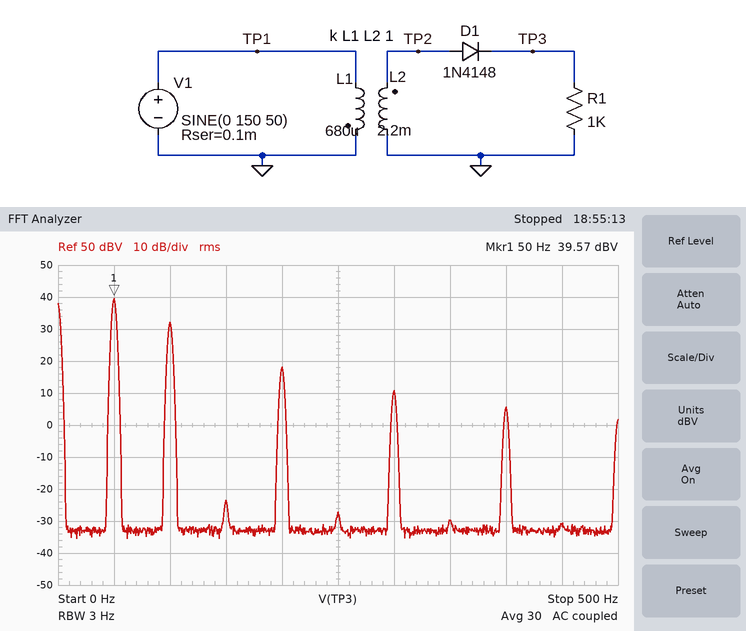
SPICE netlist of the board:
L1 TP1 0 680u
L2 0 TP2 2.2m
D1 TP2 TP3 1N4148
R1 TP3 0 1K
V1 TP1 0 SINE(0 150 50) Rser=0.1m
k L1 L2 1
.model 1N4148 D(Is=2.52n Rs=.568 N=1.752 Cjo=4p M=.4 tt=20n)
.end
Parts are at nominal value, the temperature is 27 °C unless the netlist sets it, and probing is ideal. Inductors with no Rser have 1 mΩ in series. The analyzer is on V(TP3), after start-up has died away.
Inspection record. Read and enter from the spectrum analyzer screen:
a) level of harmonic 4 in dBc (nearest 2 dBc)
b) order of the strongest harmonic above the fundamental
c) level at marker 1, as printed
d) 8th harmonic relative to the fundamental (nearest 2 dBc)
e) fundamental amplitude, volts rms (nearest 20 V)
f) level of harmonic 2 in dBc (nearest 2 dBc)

-22 dBc
2
39.57 dBV
-34 dBc
100 V
-8 dBc
